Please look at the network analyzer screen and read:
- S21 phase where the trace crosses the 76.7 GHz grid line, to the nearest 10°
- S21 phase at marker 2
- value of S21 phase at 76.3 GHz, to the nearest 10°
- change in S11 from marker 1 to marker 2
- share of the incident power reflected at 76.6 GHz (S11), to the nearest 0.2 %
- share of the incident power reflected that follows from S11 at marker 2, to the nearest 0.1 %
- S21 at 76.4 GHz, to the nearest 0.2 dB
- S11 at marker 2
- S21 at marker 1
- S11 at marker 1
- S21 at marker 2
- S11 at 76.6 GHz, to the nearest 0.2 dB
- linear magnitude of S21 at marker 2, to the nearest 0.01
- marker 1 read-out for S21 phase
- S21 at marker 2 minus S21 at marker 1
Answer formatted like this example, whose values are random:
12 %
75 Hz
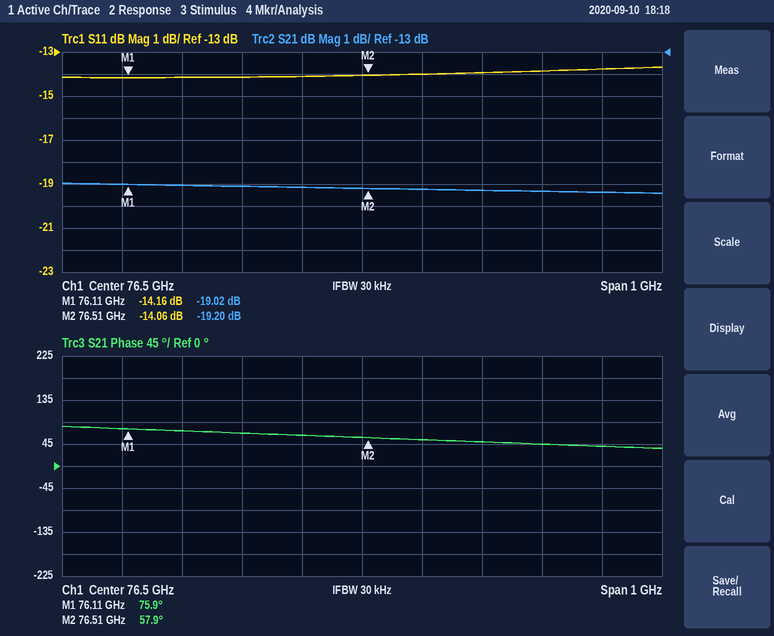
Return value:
50°
57.9°
70°
0.10 dB
4.0 %
3.9 %
-19.2 dB
-14.06 dB
-19.02 dB
-14.16 dB
-19.20 dB
-14.0 dB
0.11
75.9°
-0.18 dB
